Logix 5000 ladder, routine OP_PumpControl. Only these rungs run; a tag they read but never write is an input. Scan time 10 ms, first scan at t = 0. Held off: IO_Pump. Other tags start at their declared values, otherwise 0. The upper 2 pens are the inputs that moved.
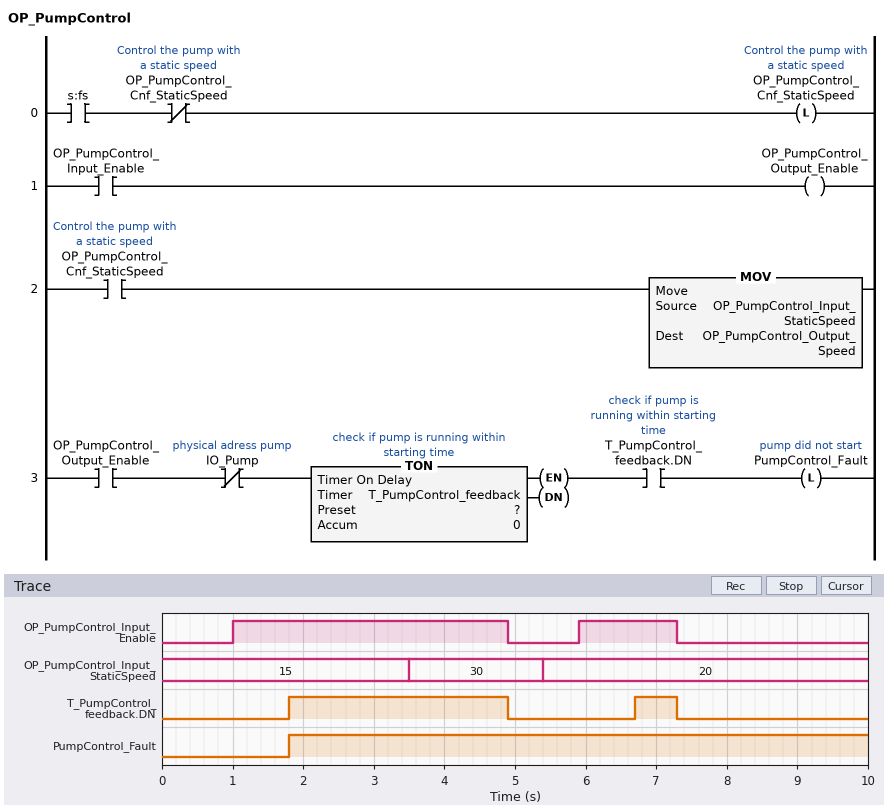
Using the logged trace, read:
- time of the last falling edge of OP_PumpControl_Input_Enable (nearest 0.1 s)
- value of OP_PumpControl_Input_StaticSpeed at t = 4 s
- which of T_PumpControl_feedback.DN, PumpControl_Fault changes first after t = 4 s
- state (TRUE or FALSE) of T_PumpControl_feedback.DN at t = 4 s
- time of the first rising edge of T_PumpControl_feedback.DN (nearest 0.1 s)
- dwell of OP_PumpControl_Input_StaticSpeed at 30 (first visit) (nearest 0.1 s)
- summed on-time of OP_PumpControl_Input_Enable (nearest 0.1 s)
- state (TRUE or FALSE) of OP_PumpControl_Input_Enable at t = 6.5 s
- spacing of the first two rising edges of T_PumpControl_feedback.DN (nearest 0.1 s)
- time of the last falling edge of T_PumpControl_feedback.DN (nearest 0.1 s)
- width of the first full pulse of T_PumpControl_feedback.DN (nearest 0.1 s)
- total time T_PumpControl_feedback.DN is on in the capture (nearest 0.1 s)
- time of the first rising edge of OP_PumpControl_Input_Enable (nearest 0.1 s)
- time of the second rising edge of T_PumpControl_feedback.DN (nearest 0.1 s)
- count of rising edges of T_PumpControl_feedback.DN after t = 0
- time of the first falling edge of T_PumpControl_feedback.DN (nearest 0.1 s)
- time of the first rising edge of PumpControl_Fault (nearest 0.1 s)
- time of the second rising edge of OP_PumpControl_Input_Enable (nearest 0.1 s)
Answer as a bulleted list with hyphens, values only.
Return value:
- 7.3 s
- 30
- T_PumpControl_feedback.DN
- TRUE
- 1.8 s
- 1.9 s
- 5.3 s
- TRUE
- 4.9 s
- 7.3 s
- 3.1 s
- 3.7 s
- 1.0 s
- 6.7 s
- 2
- 4.9 s
- 1.8 s
- 5.9 s
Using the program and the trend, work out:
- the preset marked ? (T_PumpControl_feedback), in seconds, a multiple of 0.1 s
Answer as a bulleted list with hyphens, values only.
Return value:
- 0.8 s
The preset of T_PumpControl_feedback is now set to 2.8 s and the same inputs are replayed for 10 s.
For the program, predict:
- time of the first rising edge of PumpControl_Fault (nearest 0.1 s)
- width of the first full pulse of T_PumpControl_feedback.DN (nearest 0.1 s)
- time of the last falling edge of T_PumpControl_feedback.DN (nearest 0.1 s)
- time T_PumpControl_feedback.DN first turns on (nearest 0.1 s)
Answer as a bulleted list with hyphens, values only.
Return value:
- 3.8 s
- 1.1 s
- 4.9 s
- 3.8 s
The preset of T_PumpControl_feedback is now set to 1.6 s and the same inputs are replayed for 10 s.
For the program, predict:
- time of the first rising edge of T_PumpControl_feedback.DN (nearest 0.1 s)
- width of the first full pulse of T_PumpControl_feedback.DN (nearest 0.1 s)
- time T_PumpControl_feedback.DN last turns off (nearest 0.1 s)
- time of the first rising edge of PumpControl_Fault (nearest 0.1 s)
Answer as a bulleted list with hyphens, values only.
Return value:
- 2.6 s
- 2.3 s
- 4.9 s
- 2.6 s
